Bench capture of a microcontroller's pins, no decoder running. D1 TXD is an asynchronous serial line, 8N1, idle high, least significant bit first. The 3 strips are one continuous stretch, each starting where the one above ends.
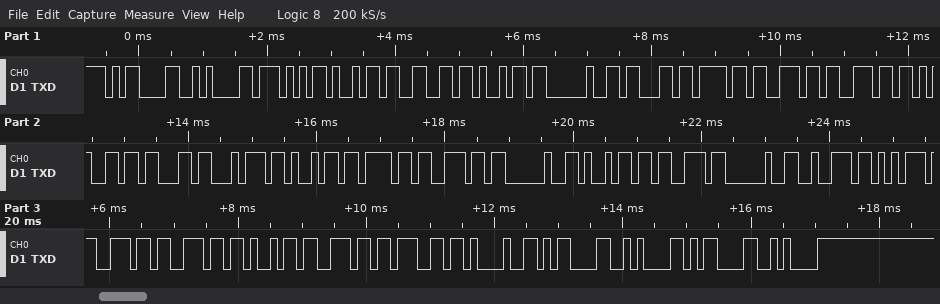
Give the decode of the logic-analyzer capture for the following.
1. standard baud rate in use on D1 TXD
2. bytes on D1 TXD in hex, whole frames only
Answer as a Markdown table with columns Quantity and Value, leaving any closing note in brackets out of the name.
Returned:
| Quantity | Value |
|---|---|
| standard baud rate in use on D1 TXD | 9600 baud |
| bytes on D1 TXD in hex, whole frames only | 0x0D 0x0A 0x57 0x69 0x66 0x69 0x20 0x63 0x6F 0x6E 0x6E 0x65 0x63 0x74 0x69 0x6F 0x6E 0x20 0x69 0x73 0x20 0x72 0x75 0x6E 0x6E 0x69 0x6E 0x67 0x21 0x0D 0x0A 0x0D 0x0A |
